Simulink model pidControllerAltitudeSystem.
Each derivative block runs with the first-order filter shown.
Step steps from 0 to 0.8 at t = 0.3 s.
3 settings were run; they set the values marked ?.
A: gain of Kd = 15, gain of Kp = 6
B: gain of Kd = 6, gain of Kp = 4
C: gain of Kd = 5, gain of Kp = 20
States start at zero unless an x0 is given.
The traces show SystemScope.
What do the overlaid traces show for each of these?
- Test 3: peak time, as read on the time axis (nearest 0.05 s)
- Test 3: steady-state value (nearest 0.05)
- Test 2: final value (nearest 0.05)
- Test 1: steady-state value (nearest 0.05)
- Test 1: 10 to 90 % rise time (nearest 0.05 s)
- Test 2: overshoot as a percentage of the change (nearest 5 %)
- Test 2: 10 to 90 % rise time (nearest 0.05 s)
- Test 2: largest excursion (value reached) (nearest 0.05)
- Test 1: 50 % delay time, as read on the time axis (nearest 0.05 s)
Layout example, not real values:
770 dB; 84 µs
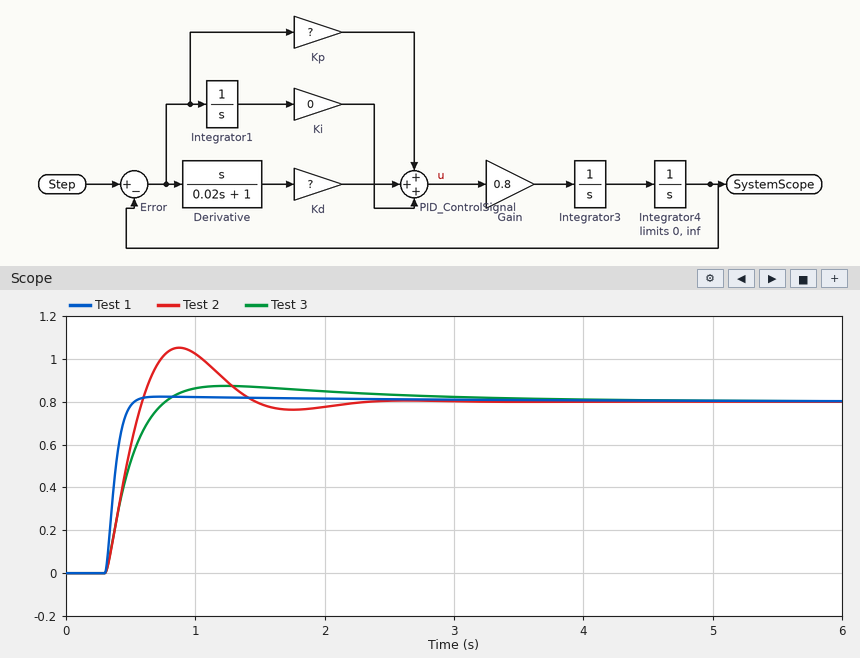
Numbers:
1.25 s; 0.80; 0.80; 0.80; 0.15 s; 30 %; 0.20 s; 1.05; 0.35 s
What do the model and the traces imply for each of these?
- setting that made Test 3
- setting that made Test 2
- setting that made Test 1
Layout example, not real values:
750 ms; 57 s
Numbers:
B; C; A
